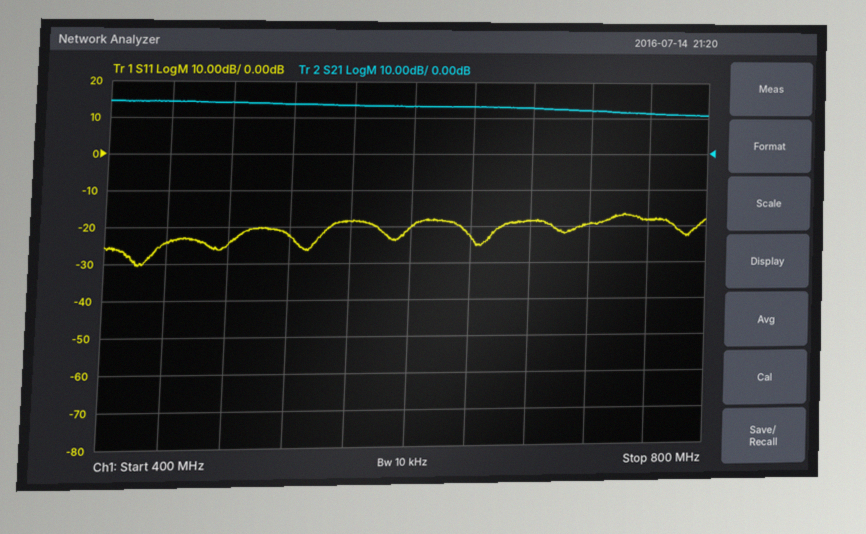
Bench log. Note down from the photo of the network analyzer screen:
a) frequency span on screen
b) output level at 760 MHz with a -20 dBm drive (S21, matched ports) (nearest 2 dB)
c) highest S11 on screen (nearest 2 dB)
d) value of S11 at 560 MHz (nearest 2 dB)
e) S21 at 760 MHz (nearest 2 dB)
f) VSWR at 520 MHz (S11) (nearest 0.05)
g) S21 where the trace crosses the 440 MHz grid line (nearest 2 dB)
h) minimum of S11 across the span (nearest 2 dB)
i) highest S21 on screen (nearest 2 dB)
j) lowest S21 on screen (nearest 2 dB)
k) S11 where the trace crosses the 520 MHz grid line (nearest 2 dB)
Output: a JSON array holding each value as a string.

["400 MHz", "-8 dBm", "-16 dB", "-18 dB", "12 dB", "1.15", "14 dB", "-30 dB", "14 dB", "10 dB", "-22 dB"]
